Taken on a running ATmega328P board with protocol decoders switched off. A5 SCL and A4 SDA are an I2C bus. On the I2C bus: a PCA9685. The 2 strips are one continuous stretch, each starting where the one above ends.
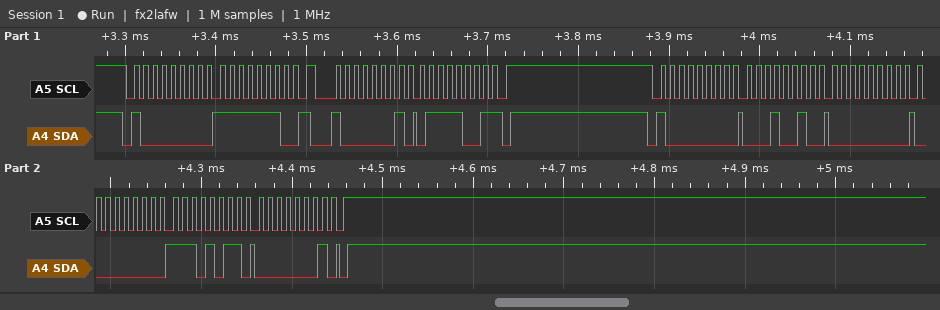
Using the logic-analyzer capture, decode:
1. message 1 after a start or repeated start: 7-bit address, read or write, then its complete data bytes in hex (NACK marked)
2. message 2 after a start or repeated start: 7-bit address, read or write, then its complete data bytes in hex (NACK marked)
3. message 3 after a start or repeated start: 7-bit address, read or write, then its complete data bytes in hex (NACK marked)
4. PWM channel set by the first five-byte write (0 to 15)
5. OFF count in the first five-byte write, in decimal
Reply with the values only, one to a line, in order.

0x40 write: FE
0x40 read: 79 NACK
0x40 write: 12 00 00 EB 01
3
491
